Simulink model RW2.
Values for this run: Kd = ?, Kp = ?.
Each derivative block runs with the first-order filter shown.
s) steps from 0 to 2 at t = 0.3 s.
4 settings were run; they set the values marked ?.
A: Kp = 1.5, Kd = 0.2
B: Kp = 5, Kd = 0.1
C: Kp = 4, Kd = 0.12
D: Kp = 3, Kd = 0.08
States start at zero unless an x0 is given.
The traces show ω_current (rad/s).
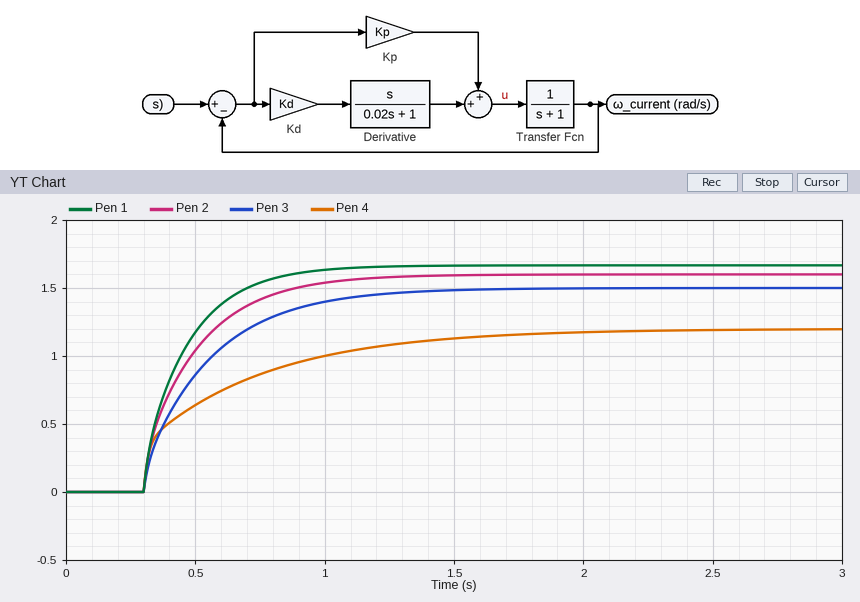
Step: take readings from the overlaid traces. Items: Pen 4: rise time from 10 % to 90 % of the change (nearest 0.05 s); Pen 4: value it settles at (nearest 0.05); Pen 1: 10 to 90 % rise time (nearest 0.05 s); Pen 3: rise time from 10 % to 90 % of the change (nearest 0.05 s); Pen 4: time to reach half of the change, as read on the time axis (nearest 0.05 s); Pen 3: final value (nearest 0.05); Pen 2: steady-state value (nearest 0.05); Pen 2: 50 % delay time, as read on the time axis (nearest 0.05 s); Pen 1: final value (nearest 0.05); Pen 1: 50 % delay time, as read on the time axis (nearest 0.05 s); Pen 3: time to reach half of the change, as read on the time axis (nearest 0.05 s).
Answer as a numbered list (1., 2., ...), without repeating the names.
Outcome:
1. 0.95 s
2. 1.20
3. 0.40 s
4. 0.60 s
5. 0.45 s
6. 1.50
7. 1.60
8. 0.40 s
9. 1.65
10. 0.40 s
11. 0.45 s
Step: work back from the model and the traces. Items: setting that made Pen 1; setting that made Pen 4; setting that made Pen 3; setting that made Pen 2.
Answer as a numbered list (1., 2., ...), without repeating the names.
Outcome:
1. B
2. A
3. D
4. C
